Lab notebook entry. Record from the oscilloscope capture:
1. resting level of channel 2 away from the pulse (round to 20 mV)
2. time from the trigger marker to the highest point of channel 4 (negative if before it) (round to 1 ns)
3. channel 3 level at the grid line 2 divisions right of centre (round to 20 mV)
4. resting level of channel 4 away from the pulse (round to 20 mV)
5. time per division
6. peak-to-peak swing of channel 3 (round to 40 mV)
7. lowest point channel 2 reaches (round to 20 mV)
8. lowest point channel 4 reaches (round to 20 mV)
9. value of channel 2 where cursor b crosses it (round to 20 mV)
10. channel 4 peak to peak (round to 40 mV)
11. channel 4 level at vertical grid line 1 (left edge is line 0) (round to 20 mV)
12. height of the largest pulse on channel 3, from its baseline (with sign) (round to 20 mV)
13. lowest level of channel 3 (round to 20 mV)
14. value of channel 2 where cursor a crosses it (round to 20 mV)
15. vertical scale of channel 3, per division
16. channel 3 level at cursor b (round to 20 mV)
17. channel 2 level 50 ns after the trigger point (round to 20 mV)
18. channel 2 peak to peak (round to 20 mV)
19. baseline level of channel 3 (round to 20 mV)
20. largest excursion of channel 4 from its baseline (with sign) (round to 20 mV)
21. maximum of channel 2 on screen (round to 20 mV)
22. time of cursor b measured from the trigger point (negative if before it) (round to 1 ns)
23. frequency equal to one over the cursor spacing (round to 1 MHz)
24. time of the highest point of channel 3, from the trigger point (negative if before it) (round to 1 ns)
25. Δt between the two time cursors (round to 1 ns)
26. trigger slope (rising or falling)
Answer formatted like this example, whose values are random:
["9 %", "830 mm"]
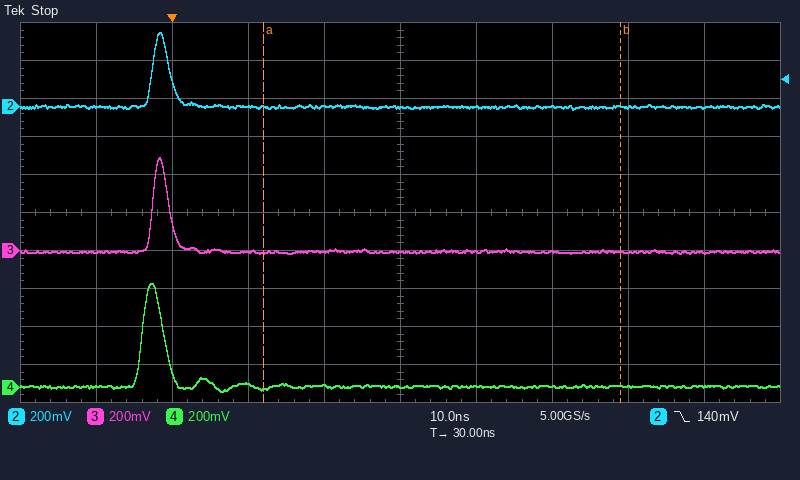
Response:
["0 mV", "-3 ns", "0 mV", "0 mV", "10 ns", "520 mV", "-20 mV", "-20 mV", "0 mV", "560 mV", "0 mV", "+500 mV", "-20 mV", "0 mV", "200 mV", "0 mV", "0 mV", "400 mV", "0 mV", "+540 mV", "380 mV", "+59 ns", "21 MHz", "-2 ns", "47 ns", "falling"]
